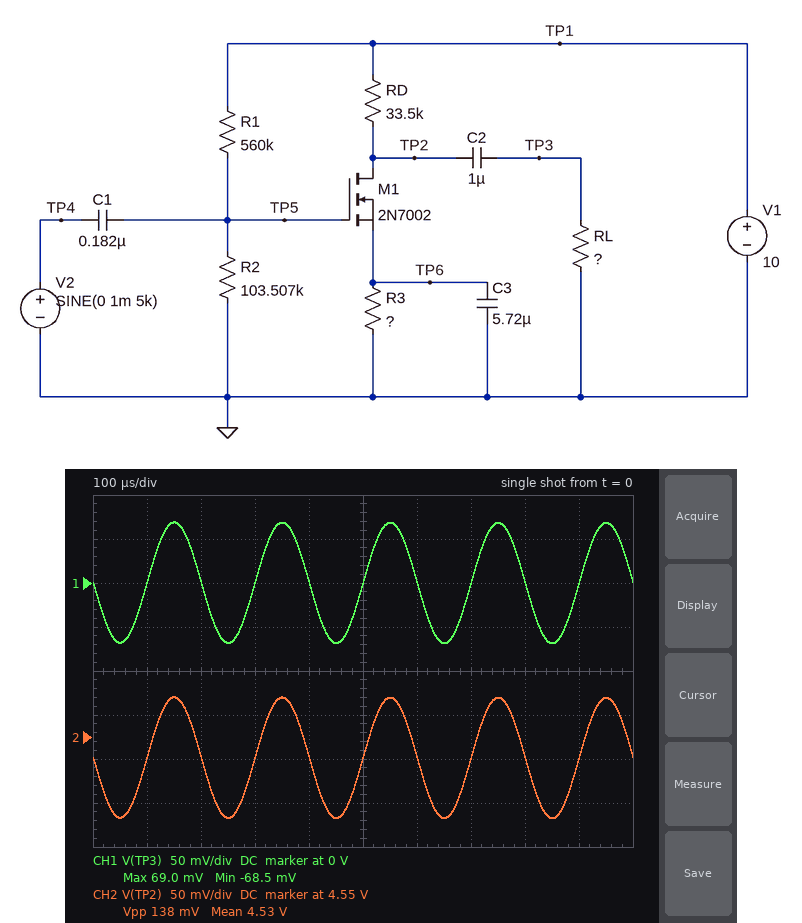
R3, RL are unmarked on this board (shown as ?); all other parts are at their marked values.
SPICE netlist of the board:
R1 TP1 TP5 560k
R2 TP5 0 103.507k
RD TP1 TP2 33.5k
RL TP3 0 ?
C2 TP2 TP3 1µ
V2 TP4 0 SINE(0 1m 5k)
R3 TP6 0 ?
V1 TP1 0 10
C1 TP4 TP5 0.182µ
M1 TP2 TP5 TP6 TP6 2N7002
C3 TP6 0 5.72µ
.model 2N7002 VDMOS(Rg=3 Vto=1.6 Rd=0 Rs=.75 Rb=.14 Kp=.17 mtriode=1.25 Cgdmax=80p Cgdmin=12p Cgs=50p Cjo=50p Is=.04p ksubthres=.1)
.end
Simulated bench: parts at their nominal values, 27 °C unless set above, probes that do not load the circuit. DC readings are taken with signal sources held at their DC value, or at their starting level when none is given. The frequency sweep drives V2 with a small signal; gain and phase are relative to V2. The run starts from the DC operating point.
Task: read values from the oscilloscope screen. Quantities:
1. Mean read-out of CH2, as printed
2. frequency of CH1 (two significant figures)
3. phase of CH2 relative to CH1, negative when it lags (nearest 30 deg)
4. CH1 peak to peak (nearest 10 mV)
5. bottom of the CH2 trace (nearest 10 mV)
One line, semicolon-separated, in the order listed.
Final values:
4.53 V; 5.0 kHz; 0 deg; 140 mV; 4.46 V
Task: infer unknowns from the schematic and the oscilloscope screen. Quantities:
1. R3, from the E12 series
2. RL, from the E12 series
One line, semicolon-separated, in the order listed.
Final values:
120 Ω; 120 kΩ
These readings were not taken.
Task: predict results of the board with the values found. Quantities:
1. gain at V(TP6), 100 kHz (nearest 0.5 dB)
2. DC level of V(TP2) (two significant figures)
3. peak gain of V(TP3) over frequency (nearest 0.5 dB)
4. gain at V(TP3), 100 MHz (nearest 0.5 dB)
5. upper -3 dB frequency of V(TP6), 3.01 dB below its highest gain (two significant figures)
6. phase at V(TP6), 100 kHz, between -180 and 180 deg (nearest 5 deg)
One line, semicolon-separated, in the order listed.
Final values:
-64.0 dB; 4.5 V; 36.5 dB; -5.5 dB; 320 Hz; -105 deg
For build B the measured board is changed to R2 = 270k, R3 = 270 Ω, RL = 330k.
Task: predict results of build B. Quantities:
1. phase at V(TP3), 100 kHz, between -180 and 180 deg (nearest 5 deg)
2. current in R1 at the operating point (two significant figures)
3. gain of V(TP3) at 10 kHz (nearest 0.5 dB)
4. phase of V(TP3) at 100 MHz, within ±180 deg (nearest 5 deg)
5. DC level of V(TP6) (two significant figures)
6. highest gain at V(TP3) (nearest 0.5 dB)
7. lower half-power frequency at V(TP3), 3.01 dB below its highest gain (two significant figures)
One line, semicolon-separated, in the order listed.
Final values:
160 deg; 12 µA; -65.5 dB; 60 deg; 80 mV; -8.5 dB; 160 MHz
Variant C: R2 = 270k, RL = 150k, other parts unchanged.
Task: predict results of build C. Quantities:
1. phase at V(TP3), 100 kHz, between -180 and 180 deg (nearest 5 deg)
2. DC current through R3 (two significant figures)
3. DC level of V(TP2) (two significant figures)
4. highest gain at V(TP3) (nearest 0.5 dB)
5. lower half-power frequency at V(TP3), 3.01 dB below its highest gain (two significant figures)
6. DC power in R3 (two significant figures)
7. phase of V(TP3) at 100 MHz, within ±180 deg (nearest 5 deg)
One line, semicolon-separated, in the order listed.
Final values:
160 deg; 300 µA; 37 mV; -8.5 dB; 160 MHz; 11 µW; 60 deg
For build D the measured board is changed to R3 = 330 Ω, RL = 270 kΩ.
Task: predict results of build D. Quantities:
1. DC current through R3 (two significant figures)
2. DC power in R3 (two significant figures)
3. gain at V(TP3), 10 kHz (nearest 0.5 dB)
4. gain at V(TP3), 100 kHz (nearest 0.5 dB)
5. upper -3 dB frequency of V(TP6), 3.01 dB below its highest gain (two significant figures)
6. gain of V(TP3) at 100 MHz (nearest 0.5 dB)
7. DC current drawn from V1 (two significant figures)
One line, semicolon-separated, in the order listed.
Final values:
120 µA; 4.6 µW; 35.5 dB; 34.0 dB; 160 Hz; -6.0 dB; 130 µA
